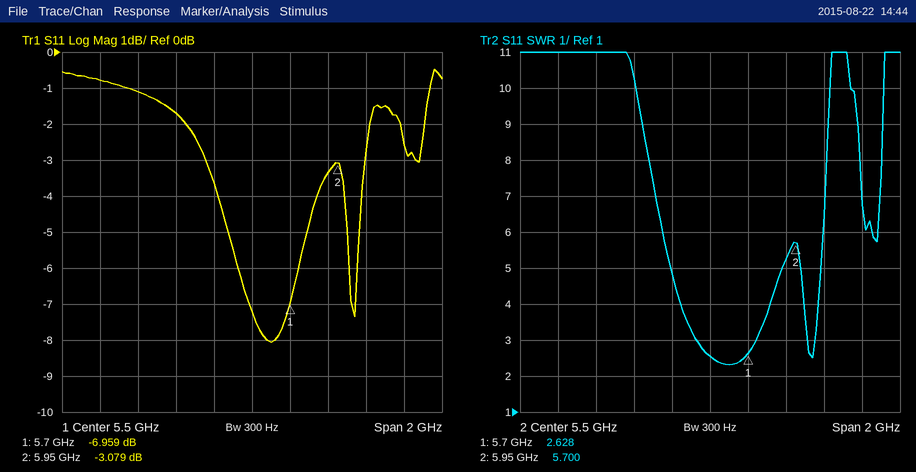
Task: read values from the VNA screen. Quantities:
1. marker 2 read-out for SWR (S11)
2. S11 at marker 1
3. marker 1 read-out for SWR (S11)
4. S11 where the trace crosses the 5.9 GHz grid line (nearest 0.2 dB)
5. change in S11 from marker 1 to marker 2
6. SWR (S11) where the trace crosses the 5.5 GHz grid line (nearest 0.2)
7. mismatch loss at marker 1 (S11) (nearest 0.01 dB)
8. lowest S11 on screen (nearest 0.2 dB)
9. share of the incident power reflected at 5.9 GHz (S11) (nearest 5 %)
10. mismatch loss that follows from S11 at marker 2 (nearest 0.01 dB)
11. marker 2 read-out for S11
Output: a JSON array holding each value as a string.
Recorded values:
["5.700", "-6.959 dB", "2.628", "-3.4 dB", "3.880 dB", "2.6", "0.98 dB", "-8.0 dB", "45 %", "2.94 dB", "-3.079 dB"]
